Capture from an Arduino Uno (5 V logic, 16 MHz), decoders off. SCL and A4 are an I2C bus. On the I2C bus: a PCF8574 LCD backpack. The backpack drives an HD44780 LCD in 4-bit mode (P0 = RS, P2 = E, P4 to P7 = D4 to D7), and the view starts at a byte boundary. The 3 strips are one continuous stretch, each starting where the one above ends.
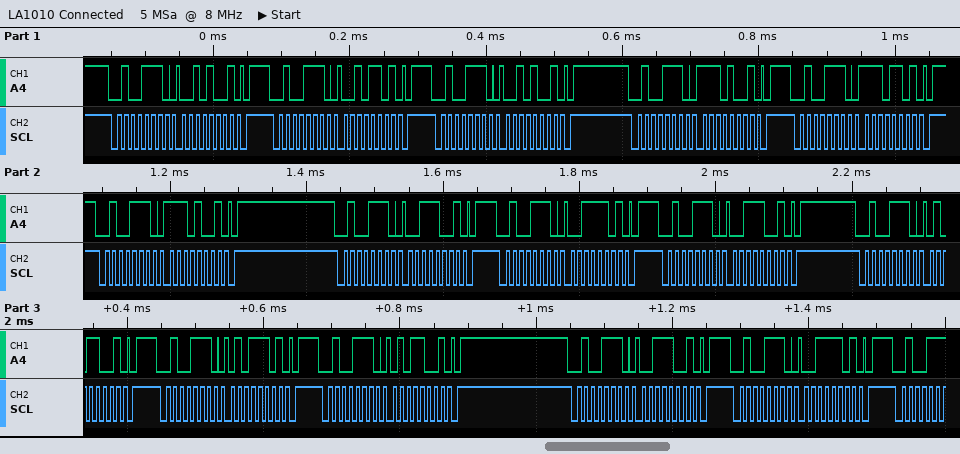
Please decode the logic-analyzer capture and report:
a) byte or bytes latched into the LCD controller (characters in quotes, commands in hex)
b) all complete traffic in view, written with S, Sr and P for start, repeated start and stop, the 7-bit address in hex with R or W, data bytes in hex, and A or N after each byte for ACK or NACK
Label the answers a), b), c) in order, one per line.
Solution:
a) '.' '5'
b) S 27W A 29 A P S 27W A 2D A P S 27W A 29 A P S 27W A E9 A P S 27W A ED A P S 27W A E9 A P S 27W A 39 A P S 27W A 3D A P S 27W A 39 A P S 27W A 59 A P S 27W A 5D A P S 27W A 59 A P S 27W A 39 A P S 27W A 3D A P
